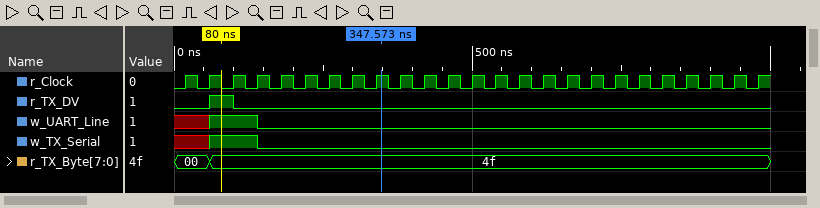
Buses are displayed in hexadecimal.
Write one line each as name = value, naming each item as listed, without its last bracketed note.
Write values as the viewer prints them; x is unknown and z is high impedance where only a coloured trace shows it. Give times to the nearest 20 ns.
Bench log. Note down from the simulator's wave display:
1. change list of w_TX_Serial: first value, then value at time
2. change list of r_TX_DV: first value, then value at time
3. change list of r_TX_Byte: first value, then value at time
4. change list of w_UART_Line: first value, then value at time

change list of w_TX_Serial: first value, then value at time = x, 1 at 60 ns, 0 at 140 ns
change list of r_TX_DV: first value, then value at time = 0, 1 at 60 ns, 0 at 100 ns
change list of r_TX_Byte: first value, then value at time = 00, 4f at 60 ns
change list of w_UART_Line: first value, then value at time = x, 1 at 60 ns, 0 at 140 ns
